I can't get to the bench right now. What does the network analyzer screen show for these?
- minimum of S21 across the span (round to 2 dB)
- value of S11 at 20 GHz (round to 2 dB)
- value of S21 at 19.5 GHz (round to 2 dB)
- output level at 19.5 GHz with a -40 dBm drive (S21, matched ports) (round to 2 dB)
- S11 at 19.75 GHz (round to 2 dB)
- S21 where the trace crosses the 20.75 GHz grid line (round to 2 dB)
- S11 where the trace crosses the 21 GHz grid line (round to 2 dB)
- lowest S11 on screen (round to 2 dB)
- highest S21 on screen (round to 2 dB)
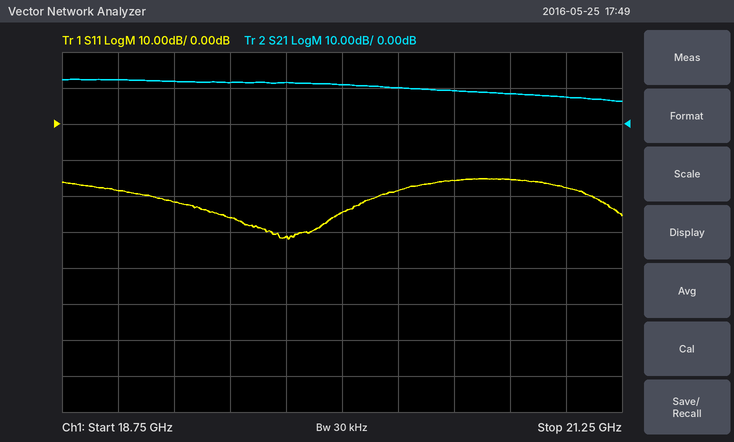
6 dB
-24 dB
12 dB
-28 dBm
-32 dB
8 dB
-18 dB
-32 dB
12 dB
